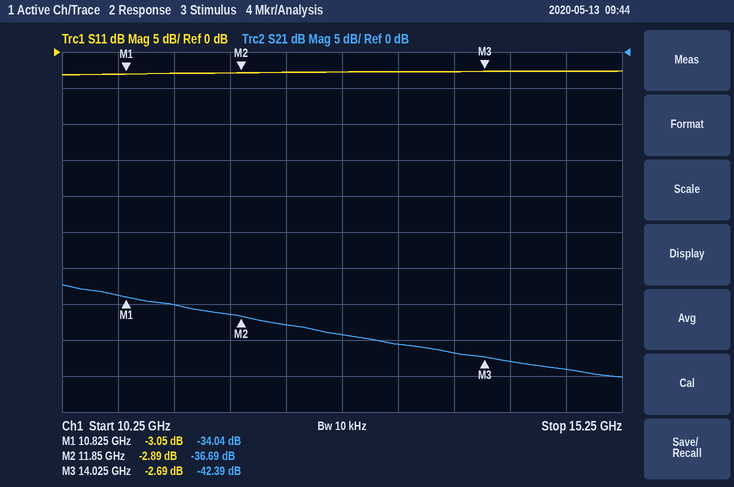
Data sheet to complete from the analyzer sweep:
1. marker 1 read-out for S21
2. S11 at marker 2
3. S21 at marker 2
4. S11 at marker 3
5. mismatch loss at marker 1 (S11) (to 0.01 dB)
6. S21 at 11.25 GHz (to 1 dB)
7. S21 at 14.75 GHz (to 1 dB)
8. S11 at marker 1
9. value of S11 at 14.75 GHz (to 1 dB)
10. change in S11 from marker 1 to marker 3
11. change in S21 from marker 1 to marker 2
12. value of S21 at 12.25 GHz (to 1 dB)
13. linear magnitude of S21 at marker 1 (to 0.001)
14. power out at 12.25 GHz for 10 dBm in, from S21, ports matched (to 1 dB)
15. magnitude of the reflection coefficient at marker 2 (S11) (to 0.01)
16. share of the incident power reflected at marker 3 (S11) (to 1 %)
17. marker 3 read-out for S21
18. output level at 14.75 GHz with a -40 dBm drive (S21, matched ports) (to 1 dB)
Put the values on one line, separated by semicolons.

-34.04 dB; -2.89 dB; -36.69 dB; -2.69 dB; 2.97 dB; -35 dB; -44 dB; -3.05 dB; -3 dB; 0.36 dB; -2.65 dB; -38 dB; 0.020; -28 dBm; 0.72; 54 %; -42.39 dB; -84 dBm
